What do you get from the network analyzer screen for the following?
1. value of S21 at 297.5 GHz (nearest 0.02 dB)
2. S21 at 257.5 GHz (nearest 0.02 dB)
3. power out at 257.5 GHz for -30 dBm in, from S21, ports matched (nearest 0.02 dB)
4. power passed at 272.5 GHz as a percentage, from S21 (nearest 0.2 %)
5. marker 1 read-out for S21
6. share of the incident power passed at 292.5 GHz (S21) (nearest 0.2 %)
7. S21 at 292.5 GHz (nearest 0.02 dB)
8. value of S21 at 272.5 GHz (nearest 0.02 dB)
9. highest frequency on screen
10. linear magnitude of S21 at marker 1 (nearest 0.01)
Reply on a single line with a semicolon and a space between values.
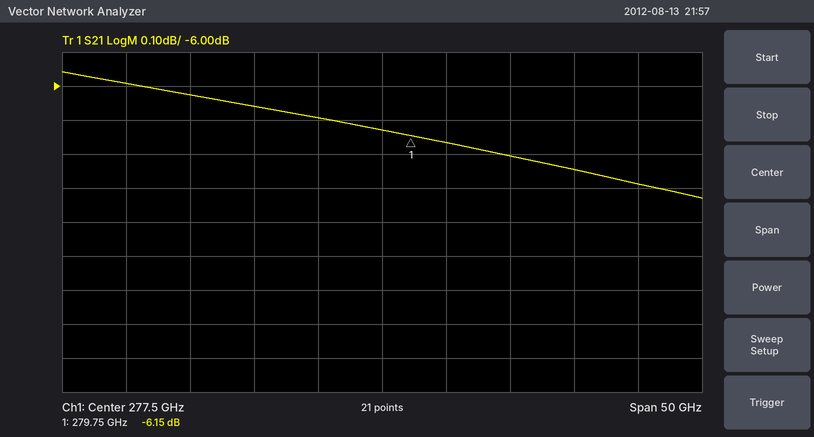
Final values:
-6.28 dB; -6.00 dB; -36.00 dBm; 24.6 %; -6.15 dB; 23.8 %; -6.24 dB; -6.10 dB; 302.5 GHz; 0.49
